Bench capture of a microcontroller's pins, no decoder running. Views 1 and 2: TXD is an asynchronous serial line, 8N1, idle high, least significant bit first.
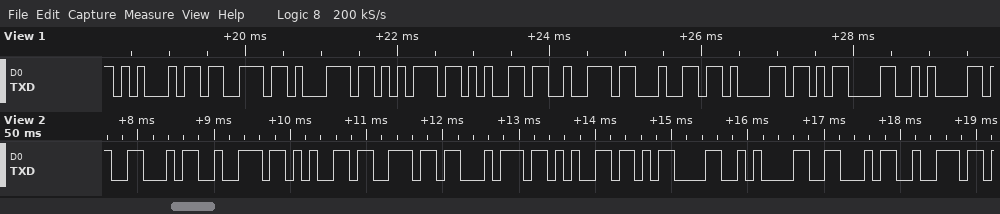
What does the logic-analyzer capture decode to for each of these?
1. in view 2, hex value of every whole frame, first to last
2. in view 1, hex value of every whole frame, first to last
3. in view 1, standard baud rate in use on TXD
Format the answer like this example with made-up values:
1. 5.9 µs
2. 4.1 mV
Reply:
1. 46 72 65 6E 74 65 0D 0A 46 72
2. 0x45 0x73 0x71 0x75 0x65 0x72 0x64 0x61 0x0D 0x0A
3. 9600 baud
